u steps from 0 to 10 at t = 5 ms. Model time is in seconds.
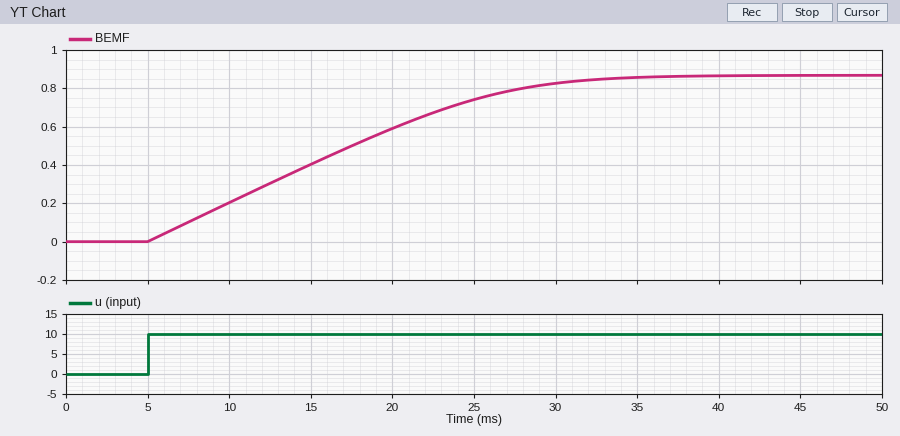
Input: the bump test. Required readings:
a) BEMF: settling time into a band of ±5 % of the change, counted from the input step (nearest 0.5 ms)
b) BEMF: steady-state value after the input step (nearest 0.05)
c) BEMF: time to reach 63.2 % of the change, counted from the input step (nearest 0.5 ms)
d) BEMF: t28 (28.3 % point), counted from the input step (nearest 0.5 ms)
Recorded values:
25.0 ms
0.85
14.0 ms
6.0 ms
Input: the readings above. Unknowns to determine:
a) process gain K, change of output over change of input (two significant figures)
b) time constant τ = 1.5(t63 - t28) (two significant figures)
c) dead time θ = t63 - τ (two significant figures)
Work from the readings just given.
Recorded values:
0.085
12 ms
2.0 ms
